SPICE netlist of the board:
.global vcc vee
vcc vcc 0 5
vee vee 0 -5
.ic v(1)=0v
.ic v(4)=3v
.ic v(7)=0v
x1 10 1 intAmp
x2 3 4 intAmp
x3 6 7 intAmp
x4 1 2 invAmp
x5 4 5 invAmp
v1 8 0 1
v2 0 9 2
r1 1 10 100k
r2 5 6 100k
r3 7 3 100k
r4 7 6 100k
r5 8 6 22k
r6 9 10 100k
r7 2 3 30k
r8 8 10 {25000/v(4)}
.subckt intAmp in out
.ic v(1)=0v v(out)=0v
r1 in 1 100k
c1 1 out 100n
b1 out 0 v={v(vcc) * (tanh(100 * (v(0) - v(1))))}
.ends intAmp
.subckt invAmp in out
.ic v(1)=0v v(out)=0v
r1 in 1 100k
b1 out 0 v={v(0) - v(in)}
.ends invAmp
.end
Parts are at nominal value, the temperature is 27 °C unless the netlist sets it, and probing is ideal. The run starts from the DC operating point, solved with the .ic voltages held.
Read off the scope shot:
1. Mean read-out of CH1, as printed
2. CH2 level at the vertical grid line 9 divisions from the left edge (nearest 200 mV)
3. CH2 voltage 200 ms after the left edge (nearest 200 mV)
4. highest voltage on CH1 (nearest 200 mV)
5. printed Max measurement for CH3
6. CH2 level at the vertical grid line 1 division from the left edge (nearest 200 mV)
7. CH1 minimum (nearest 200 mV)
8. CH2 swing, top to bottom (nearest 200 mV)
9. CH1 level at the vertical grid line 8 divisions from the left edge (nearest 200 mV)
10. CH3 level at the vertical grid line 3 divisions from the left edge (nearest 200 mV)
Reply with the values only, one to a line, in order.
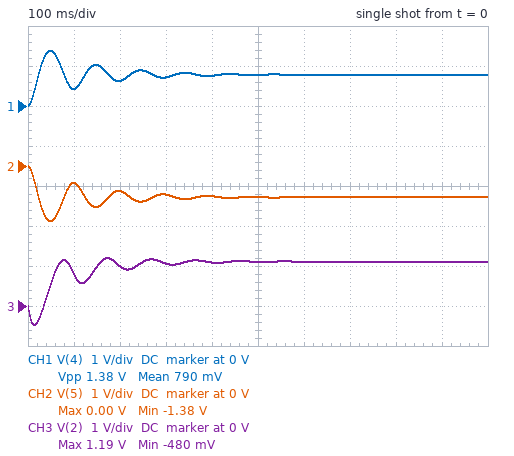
790 mV
-800 mV
-600 mV
1.4 V
1.19 V
-400 mV
0 V
1.4 V
800 mV
1.0 V
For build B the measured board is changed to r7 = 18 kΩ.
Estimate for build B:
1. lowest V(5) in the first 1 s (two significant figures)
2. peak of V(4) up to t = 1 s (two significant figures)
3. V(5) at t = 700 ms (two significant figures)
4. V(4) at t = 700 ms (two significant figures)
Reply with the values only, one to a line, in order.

-1.2 V
1.2 V
-670 mV
670 mV
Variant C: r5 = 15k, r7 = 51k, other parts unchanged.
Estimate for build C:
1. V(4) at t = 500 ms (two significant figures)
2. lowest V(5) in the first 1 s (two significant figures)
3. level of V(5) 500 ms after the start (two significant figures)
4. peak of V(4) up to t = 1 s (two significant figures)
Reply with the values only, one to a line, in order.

1.1 V
-2.0 V
-1.1 V
2.0 V
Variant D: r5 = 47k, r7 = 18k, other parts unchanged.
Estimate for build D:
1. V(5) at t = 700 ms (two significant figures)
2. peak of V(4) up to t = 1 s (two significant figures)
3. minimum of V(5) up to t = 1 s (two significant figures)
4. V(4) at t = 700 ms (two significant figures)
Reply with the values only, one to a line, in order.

-570 mV
1.1 V
-1.1 V
570 mV
